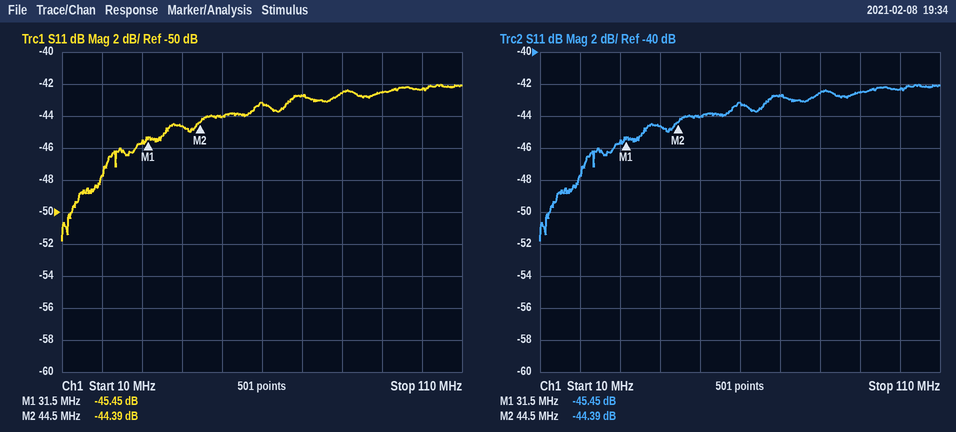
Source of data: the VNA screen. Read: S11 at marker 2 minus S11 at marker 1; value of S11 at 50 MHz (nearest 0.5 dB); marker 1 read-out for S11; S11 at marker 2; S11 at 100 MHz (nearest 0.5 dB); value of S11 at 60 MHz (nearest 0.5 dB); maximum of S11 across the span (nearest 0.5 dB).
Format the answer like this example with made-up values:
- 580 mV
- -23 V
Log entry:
- 1.06 dB
- -44.0 dB
- -45.45 dB
- -44.39 dB
- -42.5 dB
- -43.0 dB
- -42.0 dB
